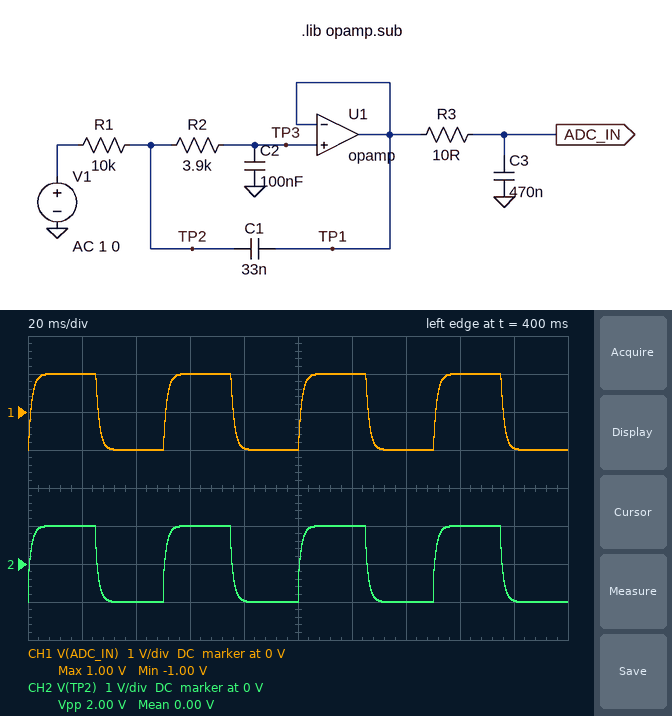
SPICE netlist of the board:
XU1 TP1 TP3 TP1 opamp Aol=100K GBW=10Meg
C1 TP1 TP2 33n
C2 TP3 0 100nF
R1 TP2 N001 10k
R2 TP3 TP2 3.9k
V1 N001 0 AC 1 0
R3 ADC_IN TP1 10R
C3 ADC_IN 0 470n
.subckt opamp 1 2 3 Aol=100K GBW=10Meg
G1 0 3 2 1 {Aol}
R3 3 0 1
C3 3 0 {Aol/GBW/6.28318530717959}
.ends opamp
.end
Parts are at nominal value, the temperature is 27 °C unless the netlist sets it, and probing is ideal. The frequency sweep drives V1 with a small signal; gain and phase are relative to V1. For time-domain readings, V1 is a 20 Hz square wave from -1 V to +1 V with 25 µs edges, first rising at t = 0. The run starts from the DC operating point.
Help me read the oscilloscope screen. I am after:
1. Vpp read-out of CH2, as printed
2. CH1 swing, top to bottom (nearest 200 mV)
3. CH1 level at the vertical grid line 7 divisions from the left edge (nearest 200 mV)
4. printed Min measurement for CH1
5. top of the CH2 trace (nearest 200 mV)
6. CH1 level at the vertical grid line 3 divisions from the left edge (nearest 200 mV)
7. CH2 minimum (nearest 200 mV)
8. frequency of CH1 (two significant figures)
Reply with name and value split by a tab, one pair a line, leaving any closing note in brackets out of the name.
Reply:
Vpp read-out of CH2, as printed	2.00 V
CH1 swing, top to bottom	2.0 V
CH1 level at the vertical grid line 7 divisions from the left edge	-1.0 V
printed Min measurement for CH1	-1.00 V
top of the CH2 trace	1.0 V
CH1 level at the vertical grid line 3 divisions from the left edge	1.0 V
CH2 minimum	-1.0 V
frequency of CH1	20 Hz
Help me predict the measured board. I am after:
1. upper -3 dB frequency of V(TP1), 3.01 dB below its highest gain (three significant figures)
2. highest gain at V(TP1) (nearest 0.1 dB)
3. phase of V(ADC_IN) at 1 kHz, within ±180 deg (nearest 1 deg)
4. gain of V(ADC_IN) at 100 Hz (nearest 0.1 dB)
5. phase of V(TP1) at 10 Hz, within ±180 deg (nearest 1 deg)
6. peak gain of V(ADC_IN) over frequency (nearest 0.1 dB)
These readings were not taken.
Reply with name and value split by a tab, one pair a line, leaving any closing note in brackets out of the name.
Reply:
upper -3 dB frequency of V(TP1), 3.01 dB below its highest gain	123 Hz
highest gain at V(TP1)	0 dB
phase of V(ADC_IN) at 1 kHz, within ±180 deg	-117 deg
gain of V(ADC_IN) at 100 Hz	-2.2 dB
phase of V(TP1) at 10 Hz, within ±180 deg	-5 deg
peak gain of V(ADC_IN) over frequency	0 dB
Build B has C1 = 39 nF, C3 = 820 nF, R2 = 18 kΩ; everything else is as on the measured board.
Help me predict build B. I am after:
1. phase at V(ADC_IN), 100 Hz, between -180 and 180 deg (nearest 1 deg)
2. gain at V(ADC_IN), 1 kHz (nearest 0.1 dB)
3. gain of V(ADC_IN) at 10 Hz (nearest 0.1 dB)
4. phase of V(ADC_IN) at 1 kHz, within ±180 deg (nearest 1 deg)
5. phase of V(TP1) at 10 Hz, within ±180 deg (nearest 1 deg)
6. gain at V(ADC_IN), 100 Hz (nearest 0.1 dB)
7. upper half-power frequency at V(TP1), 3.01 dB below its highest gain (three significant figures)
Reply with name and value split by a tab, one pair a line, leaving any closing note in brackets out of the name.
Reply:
phase at V(ADC_IN), 100 Hz, between -180 and 180 deg	-68 deg
gain at V(ADC_IN), 1 kHz	-30.1 dB
gain of V(ADC_IN) at 10 Hz	-0.1 dB
phase of V(ADC_IN) at 1 kHz, within ±180 deg	-150 deg
phase of V(TP1) at 10 Hz, within ±180 deg	-10 deg
gain at V(ADC_IN), 100 Hz	-5.6 dB
upper half-power frequency at V(TP1), 3.01 dB below its highest gain	62.4 Hz
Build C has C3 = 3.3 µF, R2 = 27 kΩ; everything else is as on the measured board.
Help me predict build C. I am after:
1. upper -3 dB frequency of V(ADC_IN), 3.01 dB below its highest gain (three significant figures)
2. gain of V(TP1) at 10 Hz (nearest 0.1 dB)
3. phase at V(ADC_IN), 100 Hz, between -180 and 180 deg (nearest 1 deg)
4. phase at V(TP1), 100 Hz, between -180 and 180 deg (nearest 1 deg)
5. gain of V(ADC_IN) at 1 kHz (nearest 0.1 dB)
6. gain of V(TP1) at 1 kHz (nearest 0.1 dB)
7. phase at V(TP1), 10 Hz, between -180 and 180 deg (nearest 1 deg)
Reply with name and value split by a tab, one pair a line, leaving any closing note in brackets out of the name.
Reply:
upper -3 dB frequency of V(ADC_IN), 3.01 dB below its highest gain	46.0 Hz
gain of V(TP1) at 10 Hz	-0.2 dB
phase at V(ADC_IN), 100 Hz, between -180 and 180 deg	-76 deg
phase at V(TP1), 100 Hz, between -180 and 180 deg	-74 deg
gain of V(ADC_IN) at 1 kHz	-32.5 dB
gain of V(TP1) at 1 kHz	-32.3 dB
phase at V(TP1), 10 Hz, between -180 and 180 deg	-13 deg
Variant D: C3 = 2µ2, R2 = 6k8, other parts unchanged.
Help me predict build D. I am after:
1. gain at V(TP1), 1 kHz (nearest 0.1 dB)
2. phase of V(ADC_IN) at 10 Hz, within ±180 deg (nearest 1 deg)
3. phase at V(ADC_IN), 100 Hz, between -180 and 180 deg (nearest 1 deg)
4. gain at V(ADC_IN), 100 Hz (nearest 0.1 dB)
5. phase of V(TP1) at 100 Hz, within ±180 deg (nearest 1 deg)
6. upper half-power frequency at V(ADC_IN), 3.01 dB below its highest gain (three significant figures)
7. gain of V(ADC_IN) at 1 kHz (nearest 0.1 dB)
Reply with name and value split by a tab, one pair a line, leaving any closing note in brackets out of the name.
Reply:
gain at V(TP1), 1 kHz	-22.4 dB
phase of V(ADC_IN) at 10 Hz, within ±180 deg	-6 deg
phase at V(ADC_IN), 100 Hz, between -180 and 180 deg	-50 deg
gain at V(ADC_IN), 100 Hz	-2.9 dB
phase of V(TP1) at 100 Hz, within ±180 deg	-49 deg
upper half-power frequency at V(ADC_IN), 3.01 dB below its highest gain	103 Hz
gain of V(ADC_IN) at 1 kHz	-22.5 dB
